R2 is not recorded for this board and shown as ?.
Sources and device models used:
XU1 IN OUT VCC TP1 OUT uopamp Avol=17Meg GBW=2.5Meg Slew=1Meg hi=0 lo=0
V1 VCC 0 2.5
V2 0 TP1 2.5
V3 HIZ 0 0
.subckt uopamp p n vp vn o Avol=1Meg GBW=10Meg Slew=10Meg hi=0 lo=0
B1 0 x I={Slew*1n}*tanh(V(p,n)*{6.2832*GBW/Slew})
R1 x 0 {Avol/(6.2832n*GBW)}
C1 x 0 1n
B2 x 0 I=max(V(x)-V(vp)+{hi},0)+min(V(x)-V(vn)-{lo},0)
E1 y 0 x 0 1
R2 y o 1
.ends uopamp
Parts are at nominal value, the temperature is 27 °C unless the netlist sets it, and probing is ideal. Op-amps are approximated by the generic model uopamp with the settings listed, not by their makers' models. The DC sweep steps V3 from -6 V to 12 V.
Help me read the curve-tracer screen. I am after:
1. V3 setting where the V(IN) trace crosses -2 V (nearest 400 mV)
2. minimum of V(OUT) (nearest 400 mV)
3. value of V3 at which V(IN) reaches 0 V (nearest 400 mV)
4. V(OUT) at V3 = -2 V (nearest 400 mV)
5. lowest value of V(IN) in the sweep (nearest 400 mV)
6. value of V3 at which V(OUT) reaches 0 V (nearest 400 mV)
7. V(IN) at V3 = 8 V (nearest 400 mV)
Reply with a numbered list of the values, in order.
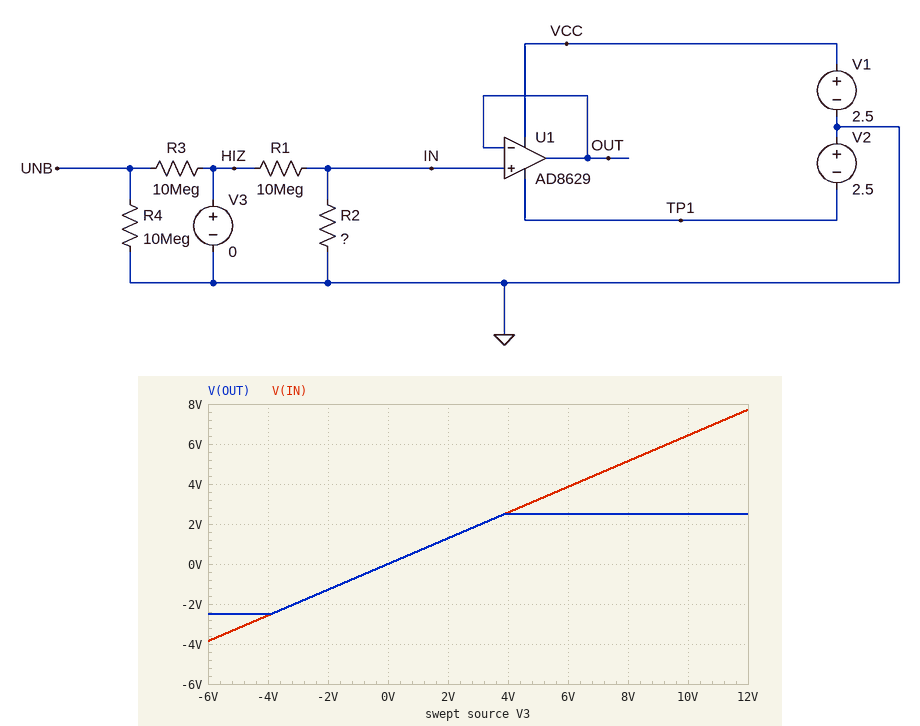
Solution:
1. -3.2 V
2. -2.4 V
3. 0 V
4. -1.2 V
5. -4.0 V
6. 0 V
7. 5.2 V
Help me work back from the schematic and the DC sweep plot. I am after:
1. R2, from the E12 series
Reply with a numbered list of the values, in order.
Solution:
1. 18 MΩ
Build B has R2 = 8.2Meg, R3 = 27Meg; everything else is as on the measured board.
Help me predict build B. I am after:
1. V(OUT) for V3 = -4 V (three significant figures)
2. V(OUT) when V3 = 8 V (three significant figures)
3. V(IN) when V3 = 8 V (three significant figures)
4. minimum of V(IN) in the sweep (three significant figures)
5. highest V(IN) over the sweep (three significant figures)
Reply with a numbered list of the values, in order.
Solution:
1. -1.80 V
2. 2.50 V
3. 3.60 V
4. -2.70 V
5. 5.41 V
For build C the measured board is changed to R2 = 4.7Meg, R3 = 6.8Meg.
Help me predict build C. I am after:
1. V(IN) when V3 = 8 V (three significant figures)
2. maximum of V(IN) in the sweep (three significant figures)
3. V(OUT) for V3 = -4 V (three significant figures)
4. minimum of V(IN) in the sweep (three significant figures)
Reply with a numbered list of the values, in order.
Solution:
1. 2.56 V
2. 3.84 V
3. -1.28 V
4. -1.92 V
